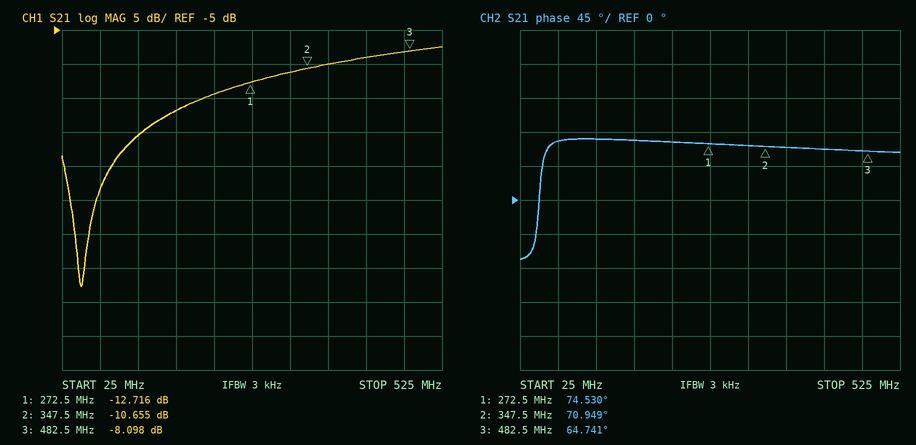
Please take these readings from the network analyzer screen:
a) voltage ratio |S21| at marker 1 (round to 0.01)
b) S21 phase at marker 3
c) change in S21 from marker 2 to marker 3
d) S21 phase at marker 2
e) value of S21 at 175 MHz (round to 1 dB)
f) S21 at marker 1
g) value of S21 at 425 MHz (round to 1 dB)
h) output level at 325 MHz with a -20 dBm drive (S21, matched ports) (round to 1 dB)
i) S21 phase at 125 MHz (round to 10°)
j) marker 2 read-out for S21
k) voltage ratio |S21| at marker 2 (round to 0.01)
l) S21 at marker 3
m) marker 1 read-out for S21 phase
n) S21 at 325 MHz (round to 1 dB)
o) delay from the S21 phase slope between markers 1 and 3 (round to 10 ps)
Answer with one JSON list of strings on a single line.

["0.23", "64.741°", "2.557 dB", "70.949°", "-17 dB", "-12.716 dB", "-9 dB", "-31 dBm", "80°", "-10.655 dB", "0.29", "-8.098 dB", "74.530°", "-11 dB", "130 ps"]
